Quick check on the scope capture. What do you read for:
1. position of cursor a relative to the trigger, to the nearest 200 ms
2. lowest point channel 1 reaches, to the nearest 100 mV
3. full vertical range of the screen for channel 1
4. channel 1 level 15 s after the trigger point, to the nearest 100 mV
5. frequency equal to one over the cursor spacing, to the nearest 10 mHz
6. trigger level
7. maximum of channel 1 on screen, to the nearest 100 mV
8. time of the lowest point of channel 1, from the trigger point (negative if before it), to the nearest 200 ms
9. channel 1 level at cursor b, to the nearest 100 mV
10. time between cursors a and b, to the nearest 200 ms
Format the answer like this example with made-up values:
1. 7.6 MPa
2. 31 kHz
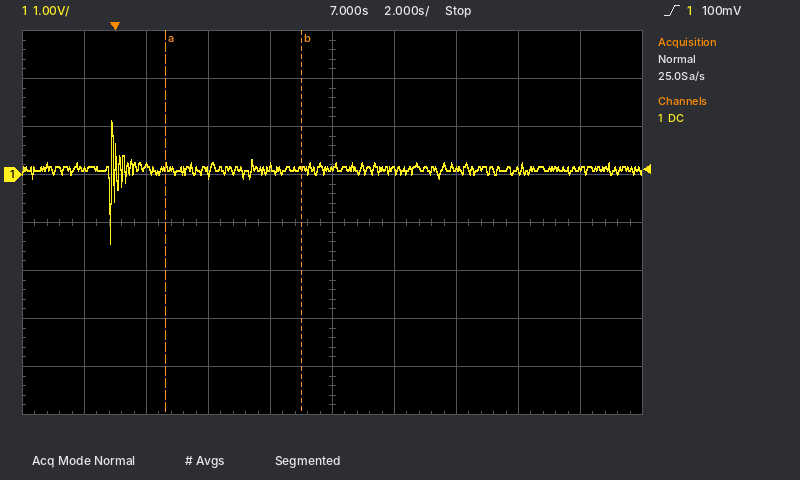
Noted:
1. +1.6 s
2. -1.4 V
3. 8 V
4. 100 mV
5. 230 mHz
6. 100 mV
7. 1.1 V
8. -200 ms
9. 100 mV
10. 4.4 s
